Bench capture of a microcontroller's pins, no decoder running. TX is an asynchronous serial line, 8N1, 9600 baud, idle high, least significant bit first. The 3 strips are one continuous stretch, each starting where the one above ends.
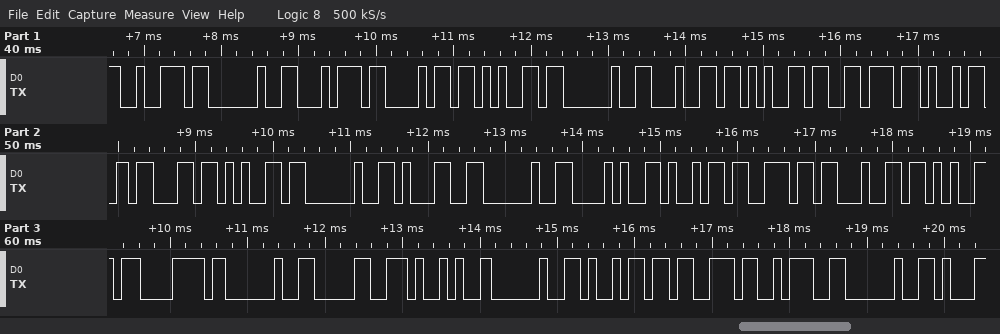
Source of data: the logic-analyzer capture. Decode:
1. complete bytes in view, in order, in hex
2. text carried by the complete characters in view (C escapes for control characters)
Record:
72 20 74 68 65 20 64 65 76 69 63 65 20 31 20 28 69 6E 64 65 78 20 30 29 20 69 73 3A 20
"r the device 1 (index 0) is: "
